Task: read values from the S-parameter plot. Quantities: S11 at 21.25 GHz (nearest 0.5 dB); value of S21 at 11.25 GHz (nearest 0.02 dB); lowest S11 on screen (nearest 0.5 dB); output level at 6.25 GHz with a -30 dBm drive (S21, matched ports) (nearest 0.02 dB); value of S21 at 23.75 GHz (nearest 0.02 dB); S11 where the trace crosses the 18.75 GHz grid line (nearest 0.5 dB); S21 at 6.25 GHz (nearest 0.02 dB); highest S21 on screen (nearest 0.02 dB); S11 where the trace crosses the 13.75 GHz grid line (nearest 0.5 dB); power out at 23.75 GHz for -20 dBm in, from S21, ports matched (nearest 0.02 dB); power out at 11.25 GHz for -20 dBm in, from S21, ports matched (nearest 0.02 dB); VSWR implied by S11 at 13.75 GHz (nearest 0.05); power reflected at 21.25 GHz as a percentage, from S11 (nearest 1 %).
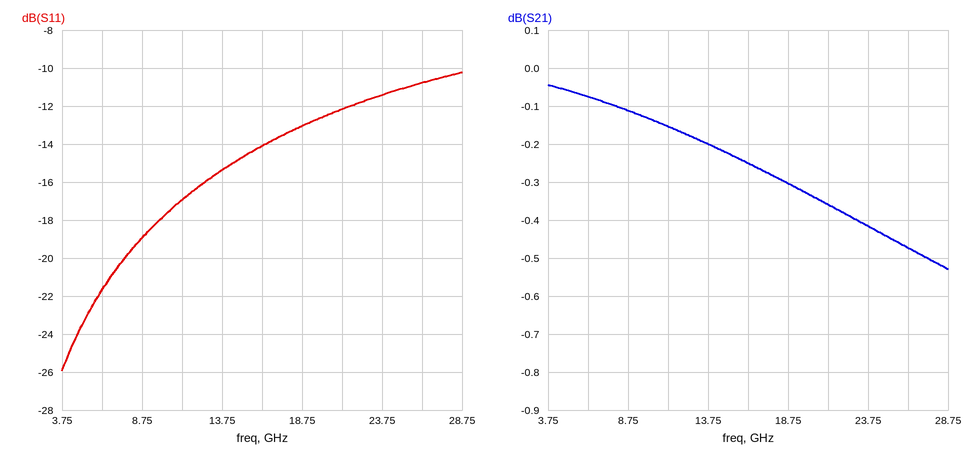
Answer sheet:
-12.0 dB
-0.16 dB
-26.0 dB
-30.08 dBm
-0.42 dB
-13.0 dB
-0.08 dB
-0.04 dB
-15.5 dB
-20.42 dBm
-20.16 dBm
1.40
6 %
